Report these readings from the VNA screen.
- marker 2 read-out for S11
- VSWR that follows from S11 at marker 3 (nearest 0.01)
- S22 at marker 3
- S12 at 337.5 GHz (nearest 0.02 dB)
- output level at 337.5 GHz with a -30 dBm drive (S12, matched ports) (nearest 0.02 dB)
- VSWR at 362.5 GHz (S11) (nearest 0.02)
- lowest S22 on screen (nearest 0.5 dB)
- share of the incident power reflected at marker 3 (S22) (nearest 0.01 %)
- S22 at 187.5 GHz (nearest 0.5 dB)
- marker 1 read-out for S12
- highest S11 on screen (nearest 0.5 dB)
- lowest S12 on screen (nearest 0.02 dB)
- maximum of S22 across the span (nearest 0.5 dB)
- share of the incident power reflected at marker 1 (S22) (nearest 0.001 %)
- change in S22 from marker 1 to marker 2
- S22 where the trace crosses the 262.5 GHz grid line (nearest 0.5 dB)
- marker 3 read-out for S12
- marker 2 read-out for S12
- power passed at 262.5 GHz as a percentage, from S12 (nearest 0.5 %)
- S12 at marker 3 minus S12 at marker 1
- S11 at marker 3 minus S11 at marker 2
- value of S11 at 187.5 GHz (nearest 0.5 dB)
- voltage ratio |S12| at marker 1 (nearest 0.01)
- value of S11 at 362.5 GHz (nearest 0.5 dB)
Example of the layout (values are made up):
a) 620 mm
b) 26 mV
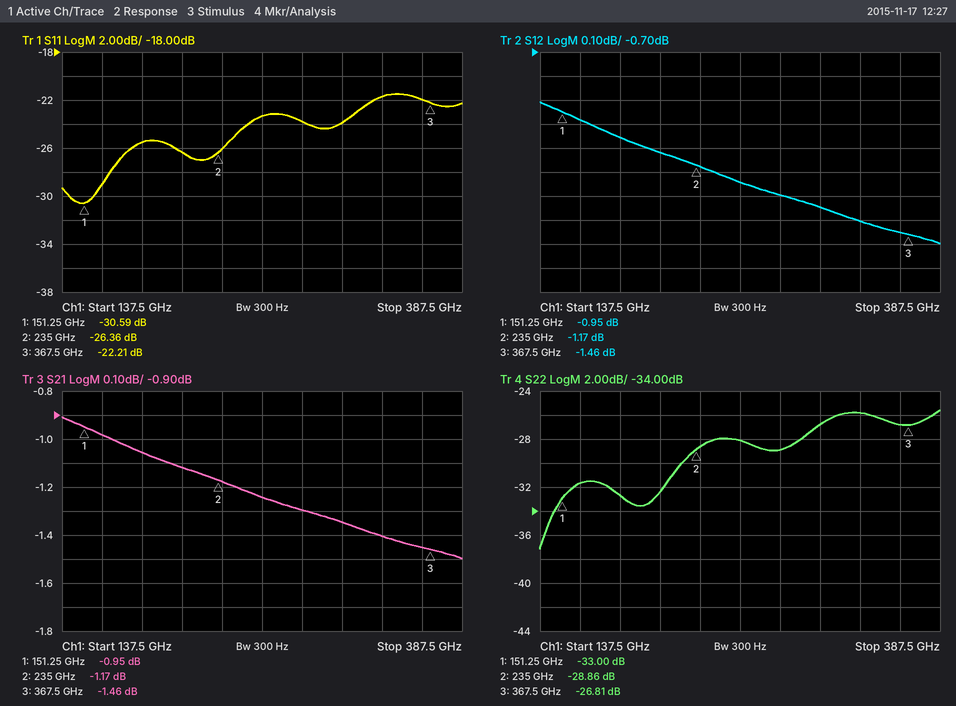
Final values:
a) -26.36 dB
b) 1.17
c) -26.81 dB
d) -1.40 dB
e) -31.40 dBm
f) 1.18
g) -37.0 dB
h) 0.21 %
i) -32.5 dB
j) -0.95 dB
k) -21.5 dB
l) -1.50 dB
m) -25.5 dB
n) 0.050 %
o) 4.14 dB
p) -28.0 dB
q) -1.46 dB
r) -1.17 dB
s) 75.0 %
t) -0.51 dB
u) 4.15 dB
v) -25.5 dB
w) 0.90
x) -22.0 dB
